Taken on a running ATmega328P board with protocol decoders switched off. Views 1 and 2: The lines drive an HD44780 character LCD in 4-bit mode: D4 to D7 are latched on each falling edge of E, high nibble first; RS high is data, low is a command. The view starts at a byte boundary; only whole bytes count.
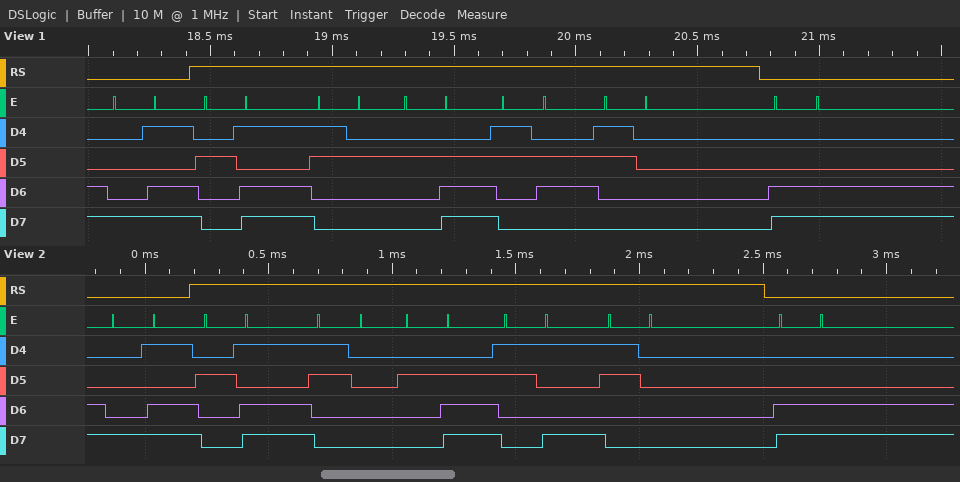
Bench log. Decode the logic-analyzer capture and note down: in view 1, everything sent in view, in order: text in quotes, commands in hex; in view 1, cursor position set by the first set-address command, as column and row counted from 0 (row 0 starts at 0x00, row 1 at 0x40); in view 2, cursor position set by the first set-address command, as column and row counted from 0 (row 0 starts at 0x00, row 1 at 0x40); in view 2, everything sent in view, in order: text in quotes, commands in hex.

0x8D "-2.60" 0xCC
column 13, row 0
column 13, row 0
0x8D "-0.90" 0xCC
